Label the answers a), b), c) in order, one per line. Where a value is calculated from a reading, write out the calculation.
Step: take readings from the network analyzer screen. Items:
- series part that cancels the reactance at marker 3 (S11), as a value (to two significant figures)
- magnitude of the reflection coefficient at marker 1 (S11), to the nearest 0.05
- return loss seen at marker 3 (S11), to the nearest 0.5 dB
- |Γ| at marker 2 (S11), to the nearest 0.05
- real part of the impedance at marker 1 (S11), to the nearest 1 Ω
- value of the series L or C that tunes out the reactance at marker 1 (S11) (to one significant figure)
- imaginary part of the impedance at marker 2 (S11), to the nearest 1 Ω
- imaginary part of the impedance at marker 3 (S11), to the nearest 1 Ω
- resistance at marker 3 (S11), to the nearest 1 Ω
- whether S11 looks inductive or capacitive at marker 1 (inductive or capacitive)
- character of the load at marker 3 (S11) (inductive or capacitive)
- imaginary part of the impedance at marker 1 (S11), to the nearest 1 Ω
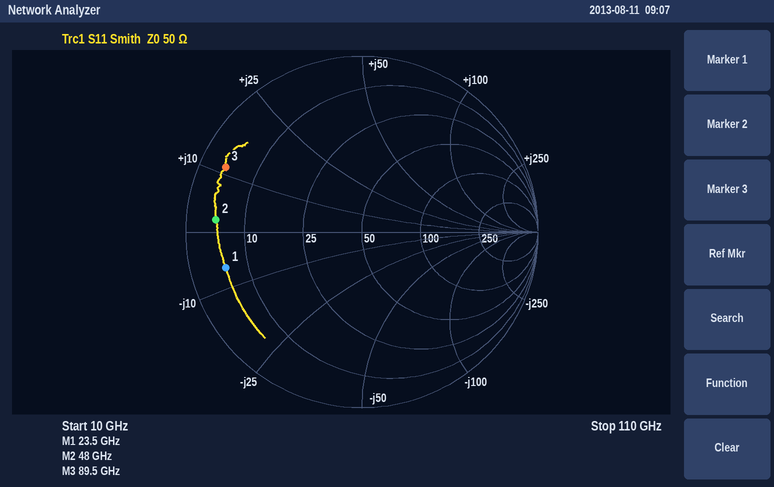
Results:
a) C = 1/(2π × 89.5 GHz × 11 Ω) ≈ 162 fF, so 160 fF to two significant figures
b) 0.80
c) 1.5 dB
d) 0.85
e) 6 Ω
f) L = 6 Ω/(2π × 23.5 GHz) ≈ 40.6 pH, so 40 pH to one significant figure
g) +2 Ω
h) +11 Ω
i) 4 Ω
j) capacitive
k) inductive
l) -6 Ω
